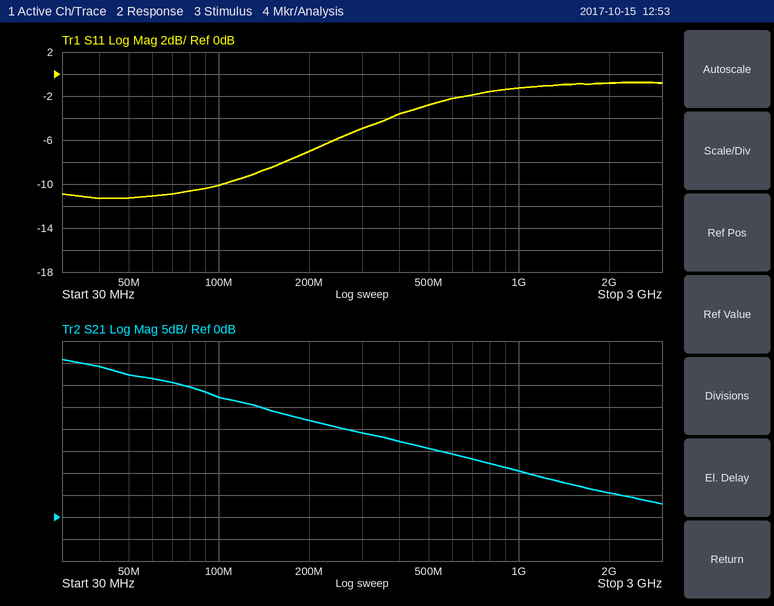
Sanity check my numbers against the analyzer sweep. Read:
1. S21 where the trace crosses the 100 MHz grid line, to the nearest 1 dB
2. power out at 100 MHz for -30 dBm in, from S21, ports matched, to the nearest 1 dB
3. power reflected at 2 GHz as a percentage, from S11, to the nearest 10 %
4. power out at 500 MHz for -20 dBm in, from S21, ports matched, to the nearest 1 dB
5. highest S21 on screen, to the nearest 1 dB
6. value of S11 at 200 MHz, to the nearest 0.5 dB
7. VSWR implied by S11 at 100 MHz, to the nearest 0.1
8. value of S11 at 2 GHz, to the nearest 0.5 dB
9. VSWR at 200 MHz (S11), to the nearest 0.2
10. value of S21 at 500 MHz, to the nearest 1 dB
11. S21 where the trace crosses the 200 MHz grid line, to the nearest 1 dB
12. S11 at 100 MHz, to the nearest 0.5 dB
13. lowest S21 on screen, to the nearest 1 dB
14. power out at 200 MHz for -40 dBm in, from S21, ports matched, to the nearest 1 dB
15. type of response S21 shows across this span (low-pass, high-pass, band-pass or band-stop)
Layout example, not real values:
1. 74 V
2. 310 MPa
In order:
1. 27 dB
2. -3 dBm
3. 80 %
4. -4 dBm
5. 36 dB
6. -7.0 dB
7. 1.9
8. -1.0 dB
9. 2.6
10. 16 dB
11. 22 dB
12. -10.0 dB
13. 3 dB
14. -18 dBm
15. low-pass
